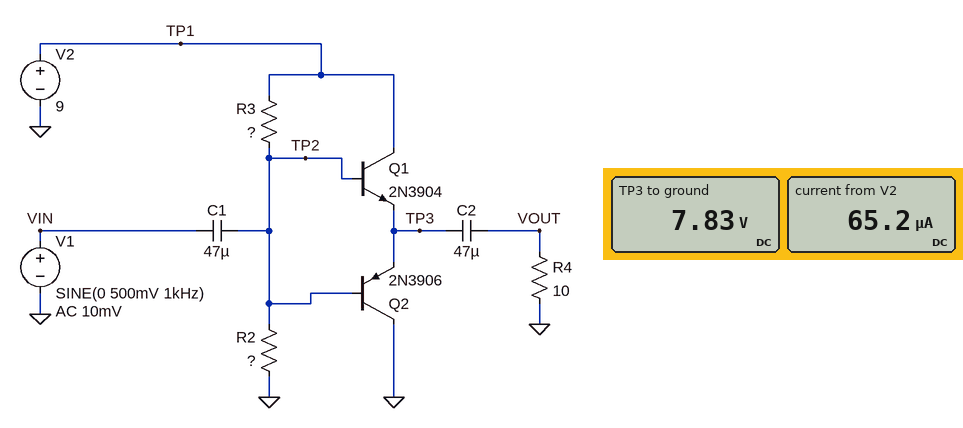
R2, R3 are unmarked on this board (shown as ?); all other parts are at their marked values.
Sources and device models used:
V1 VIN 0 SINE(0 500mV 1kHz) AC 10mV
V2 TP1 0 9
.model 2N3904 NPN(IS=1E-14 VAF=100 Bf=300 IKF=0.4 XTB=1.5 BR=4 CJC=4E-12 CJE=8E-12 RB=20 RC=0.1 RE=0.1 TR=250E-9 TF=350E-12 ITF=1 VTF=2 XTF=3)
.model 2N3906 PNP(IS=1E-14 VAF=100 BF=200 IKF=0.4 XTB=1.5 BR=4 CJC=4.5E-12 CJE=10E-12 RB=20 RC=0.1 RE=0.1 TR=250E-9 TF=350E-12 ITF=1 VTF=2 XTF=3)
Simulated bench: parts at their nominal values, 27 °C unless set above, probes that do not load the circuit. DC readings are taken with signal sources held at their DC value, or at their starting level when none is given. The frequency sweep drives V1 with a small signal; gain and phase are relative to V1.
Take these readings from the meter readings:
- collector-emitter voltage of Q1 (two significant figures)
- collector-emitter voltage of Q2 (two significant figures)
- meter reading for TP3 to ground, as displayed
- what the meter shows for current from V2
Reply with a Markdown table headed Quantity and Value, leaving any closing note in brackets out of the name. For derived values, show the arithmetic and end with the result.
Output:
| Quantity | Value |
|---|---|
| collector-emitter voltage of Q1 | 9 V - 7.83 V = 1.2 V |
| collector-emitter voltage of Q2 | 0 V - 7.83 V = -7.8 V |
| meter reading for TP3 to ground, as displayed | 7.83 V |
| what the meter shows for current from V2 | 65.2 µA |
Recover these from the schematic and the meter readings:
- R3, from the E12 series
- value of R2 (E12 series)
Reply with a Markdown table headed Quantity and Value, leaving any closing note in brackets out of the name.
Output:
| Quantity | Value |
|---|---|
| R3, from the E12 series | 18 kΩ |
| value of R2 | 120 kΩ |
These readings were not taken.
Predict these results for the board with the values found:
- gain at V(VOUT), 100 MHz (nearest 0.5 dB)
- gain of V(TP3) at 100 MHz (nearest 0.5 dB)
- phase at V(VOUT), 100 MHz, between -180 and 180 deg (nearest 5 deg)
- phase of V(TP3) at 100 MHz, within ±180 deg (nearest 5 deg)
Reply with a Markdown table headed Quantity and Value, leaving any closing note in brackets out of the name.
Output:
| Quantity | Value |
|---|---|
| gain at V(VOUT), 100 MHz | -19.0 dB |
| gain of V(TP3) at 100 MHz | -19.0 dB |
| phase at V(VOUT), 100 MHz, between -180 and 180 deg | 75 deg |
| phase of V(TP3) at 100 MHz, within ±180 deg | 75 deg |
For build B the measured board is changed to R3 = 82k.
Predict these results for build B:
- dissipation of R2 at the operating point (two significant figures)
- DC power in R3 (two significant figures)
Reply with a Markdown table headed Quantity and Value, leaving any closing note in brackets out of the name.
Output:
| Quantity | Value |
|---|---|
| dissipation of R2 at the operating point | 240 µW |
| DC power in R3 | 160 µW |
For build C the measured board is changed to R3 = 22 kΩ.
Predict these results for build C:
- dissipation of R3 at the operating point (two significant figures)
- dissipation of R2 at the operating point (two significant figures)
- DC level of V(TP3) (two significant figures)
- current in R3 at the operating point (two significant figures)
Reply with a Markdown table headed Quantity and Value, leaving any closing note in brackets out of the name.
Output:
| Quantity | Value |
|---|---|
| dissipation of R3 at the operating point | 88 µW |
| dissipation of R2 at the operating point | 480 µW |
| DC level of V(TP3) | 7.6 V |
| current in R3 at the operating point | 63 µA |
